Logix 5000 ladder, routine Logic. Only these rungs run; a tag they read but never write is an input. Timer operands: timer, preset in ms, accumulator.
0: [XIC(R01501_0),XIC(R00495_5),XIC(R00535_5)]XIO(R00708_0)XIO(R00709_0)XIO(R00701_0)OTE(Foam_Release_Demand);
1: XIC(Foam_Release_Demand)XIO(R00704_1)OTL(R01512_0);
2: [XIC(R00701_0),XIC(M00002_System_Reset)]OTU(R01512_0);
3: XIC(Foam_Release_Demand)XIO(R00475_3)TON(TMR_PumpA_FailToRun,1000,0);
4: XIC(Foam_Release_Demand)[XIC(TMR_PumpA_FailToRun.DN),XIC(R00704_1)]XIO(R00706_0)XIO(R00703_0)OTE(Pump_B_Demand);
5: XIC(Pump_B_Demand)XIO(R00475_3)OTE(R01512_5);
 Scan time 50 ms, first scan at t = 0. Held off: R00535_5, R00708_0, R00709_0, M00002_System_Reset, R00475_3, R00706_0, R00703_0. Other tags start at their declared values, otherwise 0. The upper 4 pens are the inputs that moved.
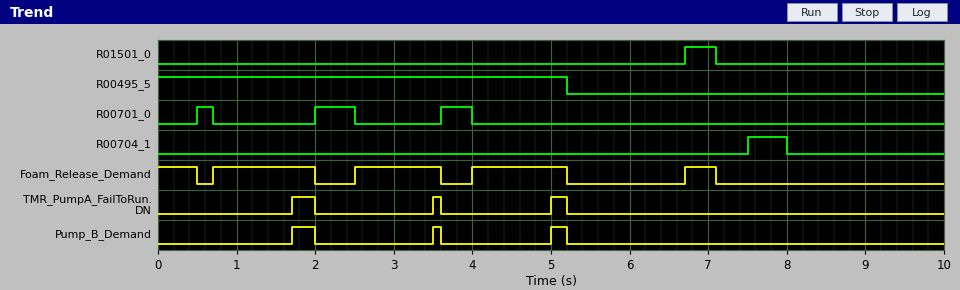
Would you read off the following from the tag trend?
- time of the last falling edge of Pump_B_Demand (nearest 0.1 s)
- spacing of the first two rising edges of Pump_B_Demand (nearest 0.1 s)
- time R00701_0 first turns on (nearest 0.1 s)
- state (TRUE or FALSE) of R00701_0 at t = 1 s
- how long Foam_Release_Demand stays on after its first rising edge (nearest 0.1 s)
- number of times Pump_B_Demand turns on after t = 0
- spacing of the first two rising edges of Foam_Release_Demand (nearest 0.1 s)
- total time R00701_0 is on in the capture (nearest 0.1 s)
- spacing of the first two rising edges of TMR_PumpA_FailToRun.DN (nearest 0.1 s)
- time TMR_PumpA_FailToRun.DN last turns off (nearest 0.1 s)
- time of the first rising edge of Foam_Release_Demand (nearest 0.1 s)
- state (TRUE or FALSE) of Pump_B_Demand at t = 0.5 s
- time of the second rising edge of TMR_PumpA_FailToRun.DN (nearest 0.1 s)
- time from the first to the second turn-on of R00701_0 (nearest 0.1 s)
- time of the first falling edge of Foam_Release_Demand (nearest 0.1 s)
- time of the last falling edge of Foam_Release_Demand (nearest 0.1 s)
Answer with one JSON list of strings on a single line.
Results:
["5.2 s", "1.8 s", "0.5 s", "FALSE", "1.3 s", "3", "1.8 s", "1.1 s", "1.8 s", "5.2 s", "0.7 s", "FALSE", "3.5 s", "1.5 s", "0.5 s", "7.1 s"]
